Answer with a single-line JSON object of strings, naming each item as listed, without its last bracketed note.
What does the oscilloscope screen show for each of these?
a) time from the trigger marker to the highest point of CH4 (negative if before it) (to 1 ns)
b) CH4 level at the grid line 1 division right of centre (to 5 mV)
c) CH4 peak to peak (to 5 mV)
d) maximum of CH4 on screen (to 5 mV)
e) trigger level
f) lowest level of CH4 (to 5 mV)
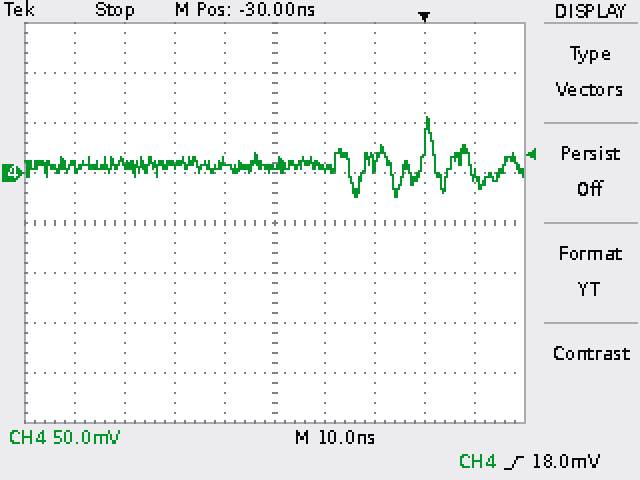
{"time from the trigger marker to the highest point of CH4 (negative if before it)": "+1 ns", "CH4 level at the grid line 1 division right of centre": "5 mV", "CH4 peak to peak": "80 mV", "maximum of CH4 on screen": "55 mV", "trigger level": "18.0 mV", "lowest level of CH4": "-25 mV"}
